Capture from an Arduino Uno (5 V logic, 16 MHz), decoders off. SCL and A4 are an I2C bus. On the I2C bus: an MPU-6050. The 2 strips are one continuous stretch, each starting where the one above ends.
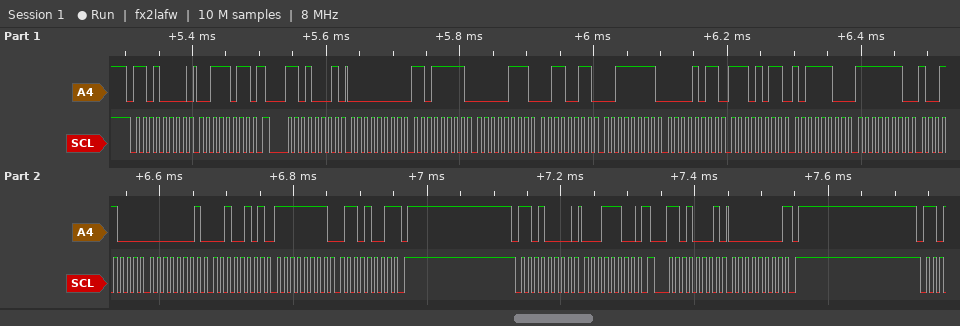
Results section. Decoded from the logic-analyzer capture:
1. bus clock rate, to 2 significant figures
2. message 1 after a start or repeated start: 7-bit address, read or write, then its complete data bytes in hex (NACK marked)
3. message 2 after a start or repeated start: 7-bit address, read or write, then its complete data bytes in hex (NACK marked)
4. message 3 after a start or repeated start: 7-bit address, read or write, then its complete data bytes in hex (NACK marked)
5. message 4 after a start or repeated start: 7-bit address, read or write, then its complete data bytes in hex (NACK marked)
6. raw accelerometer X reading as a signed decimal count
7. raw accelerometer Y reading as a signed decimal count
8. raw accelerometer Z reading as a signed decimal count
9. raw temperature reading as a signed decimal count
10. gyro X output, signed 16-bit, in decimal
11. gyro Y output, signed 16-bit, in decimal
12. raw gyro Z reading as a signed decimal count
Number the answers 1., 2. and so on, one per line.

1. 100 kHz
2. 0x68 write: 3B
3. 0x68 read: 00 DF 07 33 3F 0B EB BC FE 98 01 25 FF 69 NACK
4. 0x68 write: 1C
5. 0x68 read: 00 NACK
6. 223
7. 1843
8. 16139
9. -5188
10. -360
11. 293
12. -151
